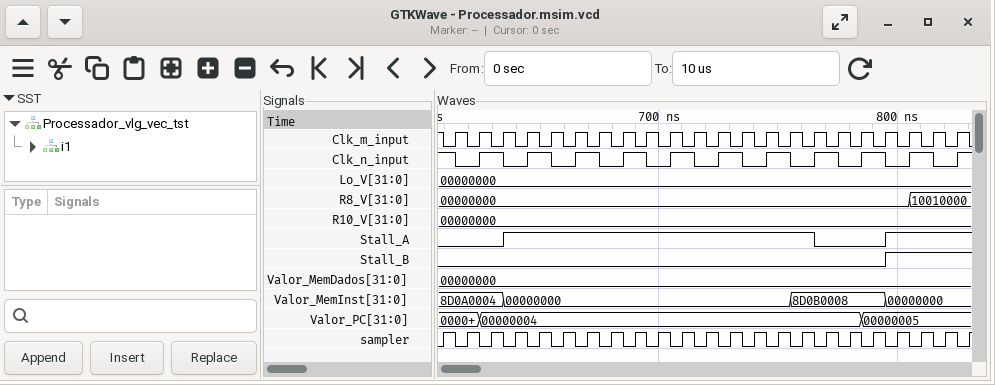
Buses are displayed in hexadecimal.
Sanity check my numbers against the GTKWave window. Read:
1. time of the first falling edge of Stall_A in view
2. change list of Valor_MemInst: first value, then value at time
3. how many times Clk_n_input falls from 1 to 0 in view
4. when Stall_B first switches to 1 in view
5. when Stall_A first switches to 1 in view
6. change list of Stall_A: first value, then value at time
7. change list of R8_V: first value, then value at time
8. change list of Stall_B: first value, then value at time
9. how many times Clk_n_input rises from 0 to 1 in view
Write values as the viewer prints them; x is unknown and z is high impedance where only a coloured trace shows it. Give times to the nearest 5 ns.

765 ns
8D0A0004, 00000000 at 635 ns, 8D0B0008 at 755 ns, 00000000 at 795 ns
11
795 ns
635 ns
0, 1 at 635 ns, 0 at 765 ns, 1 at 795 ns
00000000, 10010000 at 805 ns
0, 1 at 795 ns
11
